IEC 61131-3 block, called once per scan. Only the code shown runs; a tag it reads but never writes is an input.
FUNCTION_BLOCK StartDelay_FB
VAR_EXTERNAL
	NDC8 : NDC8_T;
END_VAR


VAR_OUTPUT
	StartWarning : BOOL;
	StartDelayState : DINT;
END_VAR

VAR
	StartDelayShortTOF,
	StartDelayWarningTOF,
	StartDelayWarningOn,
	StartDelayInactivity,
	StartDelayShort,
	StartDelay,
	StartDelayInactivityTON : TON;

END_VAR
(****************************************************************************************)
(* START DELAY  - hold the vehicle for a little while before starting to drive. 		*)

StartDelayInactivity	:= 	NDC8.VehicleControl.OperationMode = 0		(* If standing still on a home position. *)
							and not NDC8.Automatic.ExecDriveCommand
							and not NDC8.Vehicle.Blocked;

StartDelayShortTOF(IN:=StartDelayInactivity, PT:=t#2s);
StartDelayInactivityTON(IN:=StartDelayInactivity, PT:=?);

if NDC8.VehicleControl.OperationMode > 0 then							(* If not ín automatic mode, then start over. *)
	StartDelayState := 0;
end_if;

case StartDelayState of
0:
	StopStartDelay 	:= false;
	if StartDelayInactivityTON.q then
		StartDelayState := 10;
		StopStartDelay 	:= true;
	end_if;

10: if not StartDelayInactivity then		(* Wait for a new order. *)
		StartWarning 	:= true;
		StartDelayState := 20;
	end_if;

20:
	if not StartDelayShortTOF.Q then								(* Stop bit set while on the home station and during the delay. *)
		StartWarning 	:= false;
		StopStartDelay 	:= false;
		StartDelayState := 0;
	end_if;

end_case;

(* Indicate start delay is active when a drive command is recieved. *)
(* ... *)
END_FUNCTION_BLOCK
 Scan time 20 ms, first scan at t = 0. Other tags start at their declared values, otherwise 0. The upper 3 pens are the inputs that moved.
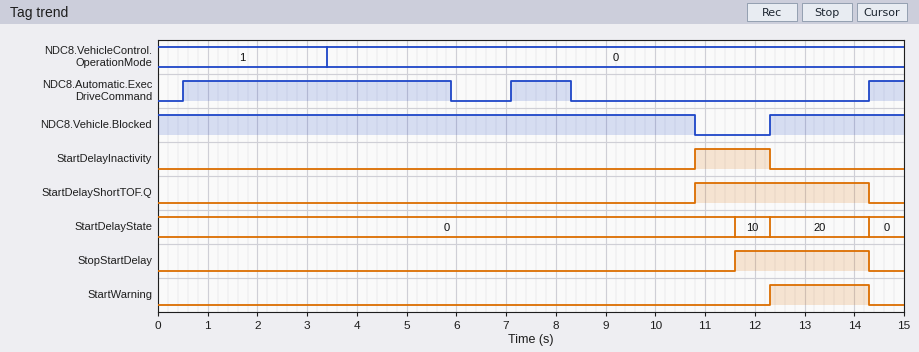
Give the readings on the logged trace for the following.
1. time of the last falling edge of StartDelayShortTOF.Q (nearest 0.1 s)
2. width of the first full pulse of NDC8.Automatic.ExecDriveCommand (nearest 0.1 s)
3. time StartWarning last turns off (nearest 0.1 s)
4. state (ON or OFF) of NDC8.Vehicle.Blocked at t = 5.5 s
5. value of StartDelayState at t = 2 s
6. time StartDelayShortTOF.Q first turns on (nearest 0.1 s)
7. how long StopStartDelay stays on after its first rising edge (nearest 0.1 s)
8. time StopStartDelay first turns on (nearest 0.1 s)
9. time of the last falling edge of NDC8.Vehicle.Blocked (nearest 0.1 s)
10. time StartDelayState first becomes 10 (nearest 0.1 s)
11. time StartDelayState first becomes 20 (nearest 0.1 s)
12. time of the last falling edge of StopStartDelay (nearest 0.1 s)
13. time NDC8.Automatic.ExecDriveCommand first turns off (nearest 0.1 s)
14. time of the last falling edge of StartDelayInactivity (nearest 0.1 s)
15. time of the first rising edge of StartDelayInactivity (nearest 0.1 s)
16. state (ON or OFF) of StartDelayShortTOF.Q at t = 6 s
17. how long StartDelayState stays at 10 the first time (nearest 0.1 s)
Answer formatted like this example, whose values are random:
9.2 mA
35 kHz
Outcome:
14.3 s
5.4 s
14.3 s
ON
0
10.8 s
2.7 s
11.6 s
10.8 s
11.6 s
12.3 s
14.3 s
5.9 s
12.3 s
10.8 s
OFF
0.7 s
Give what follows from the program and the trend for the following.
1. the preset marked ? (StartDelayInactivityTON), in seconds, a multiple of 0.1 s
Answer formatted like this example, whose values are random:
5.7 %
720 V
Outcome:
0.8 s
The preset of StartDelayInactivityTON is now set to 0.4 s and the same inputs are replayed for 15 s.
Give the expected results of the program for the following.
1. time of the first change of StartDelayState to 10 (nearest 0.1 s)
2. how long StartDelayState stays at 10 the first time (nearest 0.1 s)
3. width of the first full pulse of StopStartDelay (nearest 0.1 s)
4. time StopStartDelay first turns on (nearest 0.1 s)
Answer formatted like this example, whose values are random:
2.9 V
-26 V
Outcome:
11.2 s
1.1 s
3.1 s
11.2 s
